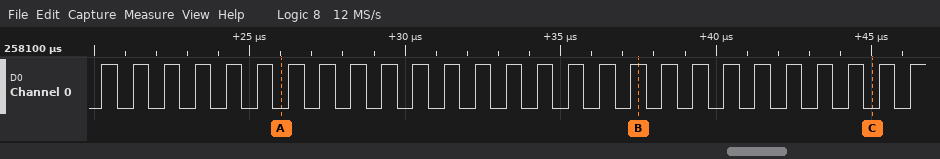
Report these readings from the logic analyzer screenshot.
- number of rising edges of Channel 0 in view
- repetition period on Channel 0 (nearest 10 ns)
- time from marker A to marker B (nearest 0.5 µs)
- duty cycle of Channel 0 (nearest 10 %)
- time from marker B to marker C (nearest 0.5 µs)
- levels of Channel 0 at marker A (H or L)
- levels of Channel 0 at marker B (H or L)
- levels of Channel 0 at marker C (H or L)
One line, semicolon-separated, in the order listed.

27; 1000 ns; 11.5 µs; 50 %; 7.5 µs; Channel 0=L; Channel 0=H; Channel 0=L
